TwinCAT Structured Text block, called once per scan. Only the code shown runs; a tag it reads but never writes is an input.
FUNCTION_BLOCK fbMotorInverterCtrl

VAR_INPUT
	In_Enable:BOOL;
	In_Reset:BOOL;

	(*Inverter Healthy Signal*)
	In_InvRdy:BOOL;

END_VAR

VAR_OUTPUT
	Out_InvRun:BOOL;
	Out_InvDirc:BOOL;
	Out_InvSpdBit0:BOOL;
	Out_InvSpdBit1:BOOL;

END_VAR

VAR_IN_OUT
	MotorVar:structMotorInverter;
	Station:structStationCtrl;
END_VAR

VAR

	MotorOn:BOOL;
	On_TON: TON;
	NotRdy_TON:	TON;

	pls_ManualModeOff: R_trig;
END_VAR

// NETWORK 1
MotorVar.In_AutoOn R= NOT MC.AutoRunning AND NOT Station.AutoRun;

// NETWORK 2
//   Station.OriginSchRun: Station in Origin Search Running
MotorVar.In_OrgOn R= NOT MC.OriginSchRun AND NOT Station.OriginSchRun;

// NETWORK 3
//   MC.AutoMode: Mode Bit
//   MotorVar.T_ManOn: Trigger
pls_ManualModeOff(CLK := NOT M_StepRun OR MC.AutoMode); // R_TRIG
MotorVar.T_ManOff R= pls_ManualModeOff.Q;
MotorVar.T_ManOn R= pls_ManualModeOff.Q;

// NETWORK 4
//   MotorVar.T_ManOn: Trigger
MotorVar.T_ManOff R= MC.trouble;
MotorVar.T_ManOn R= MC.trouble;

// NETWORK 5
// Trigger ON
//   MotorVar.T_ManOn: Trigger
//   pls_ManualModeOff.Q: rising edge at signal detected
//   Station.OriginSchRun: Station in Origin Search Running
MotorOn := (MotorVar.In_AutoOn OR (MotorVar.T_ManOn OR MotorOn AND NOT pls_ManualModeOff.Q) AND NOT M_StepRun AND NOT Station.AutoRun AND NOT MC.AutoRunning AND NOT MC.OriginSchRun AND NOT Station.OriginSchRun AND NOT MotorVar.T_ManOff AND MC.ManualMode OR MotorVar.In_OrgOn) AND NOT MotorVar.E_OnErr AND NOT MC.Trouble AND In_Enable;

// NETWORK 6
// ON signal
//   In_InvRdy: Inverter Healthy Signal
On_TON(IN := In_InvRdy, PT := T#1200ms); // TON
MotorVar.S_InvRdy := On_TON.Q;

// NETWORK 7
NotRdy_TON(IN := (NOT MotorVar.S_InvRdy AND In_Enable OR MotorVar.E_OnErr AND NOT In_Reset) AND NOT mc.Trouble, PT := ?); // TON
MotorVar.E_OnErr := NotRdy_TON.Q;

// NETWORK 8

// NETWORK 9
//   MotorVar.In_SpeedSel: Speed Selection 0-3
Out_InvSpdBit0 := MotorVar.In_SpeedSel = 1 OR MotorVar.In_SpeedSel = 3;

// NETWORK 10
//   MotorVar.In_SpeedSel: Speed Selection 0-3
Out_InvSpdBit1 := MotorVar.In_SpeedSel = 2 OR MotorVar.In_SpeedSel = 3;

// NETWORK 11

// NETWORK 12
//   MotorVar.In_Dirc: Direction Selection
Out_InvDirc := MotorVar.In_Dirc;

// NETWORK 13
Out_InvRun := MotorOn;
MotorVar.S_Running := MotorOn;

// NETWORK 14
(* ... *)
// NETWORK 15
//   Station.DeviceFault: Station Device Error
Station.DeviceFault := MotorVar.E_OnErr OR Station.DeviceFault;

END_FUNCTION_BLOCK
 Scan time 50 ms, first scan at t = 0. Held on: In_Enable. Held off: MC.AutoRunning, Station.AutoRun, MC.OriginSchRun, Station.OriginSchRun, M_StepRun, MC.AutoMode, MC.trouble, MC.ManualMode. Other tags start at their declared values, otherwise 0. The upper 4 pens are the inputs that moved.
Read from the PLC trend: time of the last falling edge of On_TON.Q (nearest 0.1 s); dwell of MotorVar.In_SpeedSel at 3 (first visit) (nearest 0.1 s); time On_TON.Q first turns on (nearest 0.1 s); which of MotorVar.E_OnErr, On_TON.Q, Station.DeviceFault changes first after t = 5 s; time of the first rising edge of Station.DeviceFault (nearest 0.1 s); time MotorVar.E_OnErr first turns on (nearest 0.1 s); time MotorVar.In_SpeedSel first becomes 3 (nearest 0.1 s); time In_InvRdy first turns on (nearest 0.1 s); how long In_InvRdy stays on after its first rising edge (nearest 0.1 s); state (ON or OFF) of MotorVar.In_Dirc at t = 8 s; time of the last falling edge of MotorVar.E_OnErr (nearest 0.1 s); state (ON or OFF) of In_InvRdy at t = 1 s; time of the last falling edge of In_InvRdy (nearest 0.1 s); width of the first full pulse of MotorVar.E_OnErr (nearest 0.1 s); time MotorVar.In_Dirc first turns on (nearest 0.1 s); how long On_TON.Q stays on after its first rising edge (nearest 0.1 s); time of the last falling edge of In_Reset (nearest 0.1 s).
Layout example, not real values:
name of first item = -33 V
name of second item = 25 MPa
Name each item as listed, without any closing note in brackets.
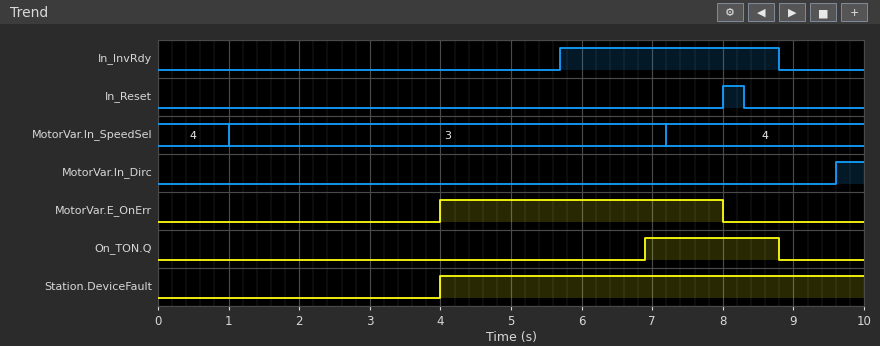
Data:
time of the last falling edge of On_TON.Q = 8.8 s
dwell of MotorVar.In_SpeedSel at 3 (first visit) = 6.2 s
time On_TON.Q first turns on = 6.9 s
which of MotorVar.E_OnErr, On_TON.Q, Station.DeviceFault changes first after t = 5 s = On_TON.Q
time of the first rising edge of Station.DeviceFault = 4.0 s
time MotorVar.E_OnErr first turns on = 4.0 s
time MotorVar.In_SpeedSel first becomes 3 = 1.0 s
time In_InvRdy first turns on = 5.7 s
how long In_InvRdy stays on after its first rising edge = 3.1 s
state (ON or OFF) of MotorVar.In_Dirc at t = 8 s = OFF
time of the last falling edge of MotorVar.E_OnErr = 8.0 s
state (ON or OFF) of In_InvRdy at t = 1 s = OFF
time of the last falling edge of In_InvRdy = 8.8 s
width of the first full pulse of MotorVar.E_OnErr = 4.0 s
time MotorVar.In_Dirc first turns on = 9.6 s
how long On_TON.Q stays on after its first rising edge = 1.9 s
time of the last falling edge of In_Reset = 8.3 s
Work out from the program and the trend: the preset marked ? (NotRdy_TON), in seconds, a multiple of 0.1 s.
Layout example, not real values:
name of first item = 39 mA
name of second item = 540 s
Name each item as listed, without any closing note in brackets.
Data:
the preset marked ? (NotRdy_TON), in seconds, a multiple of 0.1 s = 4.0 s
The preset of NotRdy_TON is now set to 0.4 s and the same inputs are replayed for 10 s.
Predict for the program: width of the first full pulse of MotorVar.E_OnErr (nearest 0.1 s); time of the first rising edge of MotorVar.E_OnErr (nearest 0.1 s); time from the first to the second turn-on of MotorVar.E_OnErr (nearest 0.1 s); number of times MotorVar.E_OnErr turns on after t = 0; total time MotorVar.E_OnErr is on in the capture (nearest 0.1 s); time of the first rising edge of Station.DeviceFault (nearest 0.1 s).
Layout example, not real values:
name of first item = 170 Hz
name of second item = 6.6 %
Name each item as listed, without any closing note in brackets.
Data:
width of the first full pulse of MotorVar.E_OnErr = 7.6 s
time of the first rising edge of MotorVar.E_OnErr = 0.4 s
time from the first to the second turn-on of MotorVar.E_OnErr = 8.8 s
number of times MotorVar.E_OnErr turns on after t = 0 = 2
total time MotorVar.E_OnErr is on in the capture = 8.4 s
time of the first rising edge of Station.DeviceFault = 0.4 s
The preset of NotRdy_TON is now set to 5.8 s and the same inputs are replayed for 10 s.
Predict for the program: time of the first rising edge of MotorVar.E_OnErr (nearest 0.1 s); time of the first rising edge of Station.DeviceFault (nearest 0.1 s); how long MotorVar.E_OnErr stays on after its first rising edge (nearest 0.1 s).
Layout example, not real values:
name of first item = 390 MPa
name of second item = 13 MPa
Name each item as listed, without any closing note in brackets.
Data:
time of the first rising edge of MotorVar.E_OnErr = 5.8 s
time of the first rising edge of Station.DeviceFault = 5.8 s
how long MotorVar.E_OnErr stays on after its first rising edge = 2.2 s
